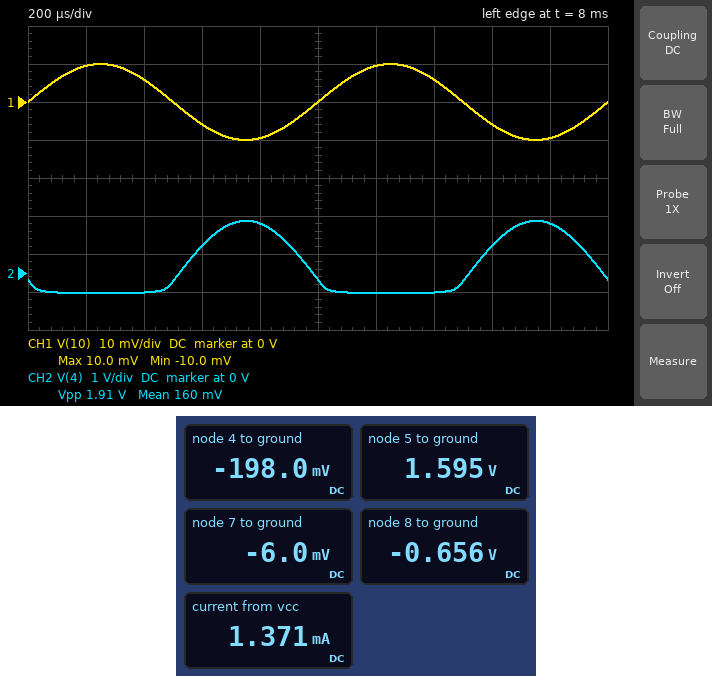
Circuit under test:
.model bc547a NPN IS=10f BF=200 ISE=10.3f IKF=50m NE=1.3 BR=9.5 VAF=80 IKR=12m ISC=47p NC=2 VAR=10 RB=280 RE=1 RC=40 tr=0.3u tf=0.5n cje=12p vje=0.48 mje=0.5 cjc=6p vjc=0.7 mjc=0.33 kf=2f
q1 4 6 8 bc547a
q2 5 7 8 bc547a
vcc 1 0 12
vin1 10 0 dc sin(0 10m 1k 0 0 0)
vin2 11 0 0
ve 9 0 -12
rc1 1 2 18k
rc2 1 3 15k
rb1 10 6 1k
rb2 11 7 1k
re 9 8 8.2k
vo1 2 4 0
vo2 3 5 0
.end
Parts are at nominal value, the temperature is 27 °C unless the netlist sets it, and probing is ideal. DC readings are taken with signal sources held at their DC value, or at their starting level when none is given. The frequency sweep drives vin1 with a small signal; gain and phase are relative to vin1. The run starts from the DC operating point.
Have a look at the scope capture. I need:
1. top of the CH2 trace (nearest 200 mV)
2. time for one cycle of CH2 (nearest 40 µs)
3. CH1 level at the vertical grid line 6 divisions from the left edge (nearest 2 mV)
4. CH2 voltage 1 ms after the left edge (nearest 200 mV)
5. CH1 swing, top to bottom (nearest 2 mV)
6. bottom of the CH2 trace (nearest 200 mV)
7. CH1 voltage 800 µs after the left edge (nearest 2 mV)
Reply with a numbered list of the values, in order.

1. 1.4 V
2. 1.00 ms
3. 10 mV
4. -200 mV
5. 20 mV
6. -600 mV
7. -10 mV
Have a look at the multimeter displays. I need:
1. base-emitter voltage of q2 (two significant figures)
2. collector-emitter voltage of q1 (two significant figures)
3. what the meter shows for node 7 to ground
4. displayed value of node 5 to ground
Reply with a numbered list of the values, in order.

1. 650 mV
2. 460 mV
3. -6.0 mV
4. 1.595 V
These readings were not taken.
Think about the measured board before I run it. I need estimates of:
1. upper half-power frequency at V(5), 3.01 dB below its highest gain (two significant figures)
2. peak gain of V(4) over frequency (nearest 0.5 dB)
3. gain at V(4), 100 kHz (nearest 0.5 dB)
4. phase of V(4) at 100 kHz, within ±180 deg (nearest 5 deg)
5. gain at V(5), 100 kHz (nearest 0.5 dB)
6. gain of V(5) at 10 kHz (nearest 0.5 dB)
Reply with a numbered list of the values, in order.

1. 74 kHz
2. 44.0 dB
3. 39.5 dB
4. 125 deg
5. 37.5 dB
6. 42.0 dB
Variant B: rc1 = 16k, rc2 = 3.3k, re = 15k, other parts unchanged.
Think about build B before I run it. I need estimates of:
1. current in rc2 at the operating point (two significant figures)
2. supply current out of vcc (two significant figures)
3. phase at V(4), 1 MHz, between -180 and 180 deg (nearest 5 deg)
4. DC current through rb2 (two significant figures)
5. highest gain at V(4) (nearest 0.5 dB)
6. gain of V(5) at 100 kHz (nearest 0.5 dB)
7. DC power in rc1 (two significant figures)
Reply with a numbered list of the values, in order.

1. 390 µA
2. 750 µA
3. 105 deg
4. 3.2 µA
5. 39.5 dB
6. 25.5 dB
7. 2.1 mW
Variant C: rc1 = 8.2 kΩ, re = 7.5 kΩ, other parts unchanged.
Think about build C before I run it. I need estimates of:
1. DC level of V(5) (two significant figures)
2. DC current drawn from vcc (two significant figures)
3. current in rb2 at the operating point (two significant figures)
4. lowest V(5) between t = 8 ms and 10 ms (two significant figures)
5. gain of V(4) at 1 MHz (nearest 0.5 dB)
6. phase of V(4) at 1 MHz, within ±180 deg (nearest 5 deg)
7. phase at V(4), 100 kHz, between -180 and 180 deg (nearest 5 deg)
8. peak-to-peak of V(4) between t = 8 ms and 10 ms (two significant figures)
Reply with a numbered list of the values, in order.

1. 1.1 V
2. 1.5 mA
3. 6.4 µA
4. -360 mV
5. 21.0 dB
6. 110 deg
7. 145 deg
8. 1.6 V
